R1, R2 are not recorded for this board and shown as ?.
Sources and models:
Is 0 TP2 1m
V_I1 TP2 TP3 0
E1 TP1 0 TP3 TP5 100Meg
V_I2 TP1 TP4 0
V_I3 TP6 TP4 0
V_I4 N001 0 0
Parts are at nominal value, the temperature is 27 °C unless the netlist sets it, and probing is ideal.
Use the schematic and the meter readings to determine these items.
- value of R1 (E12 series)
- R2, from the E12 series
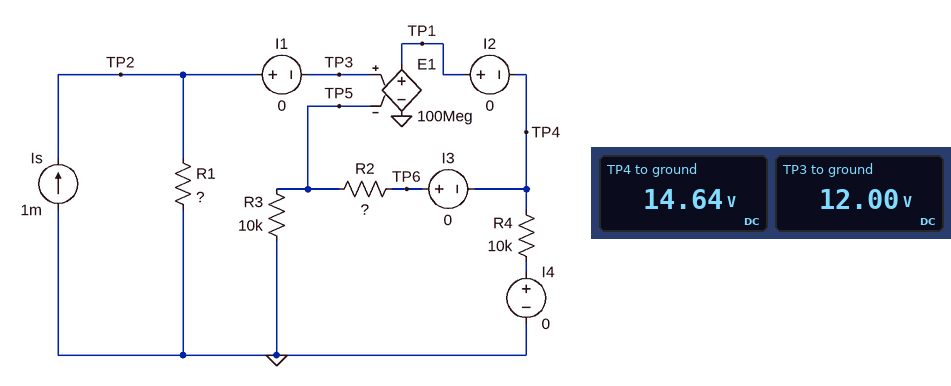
12 kΩ
2.2 kΩ
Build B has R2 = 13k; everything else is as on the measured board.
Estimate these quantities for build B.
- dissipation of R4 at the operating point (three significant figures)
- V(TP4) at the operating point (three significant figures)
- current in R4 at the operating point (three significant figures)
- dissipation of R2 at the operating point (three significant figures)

76.2 mW
27.6 V
2.76 mA
18.7 mW
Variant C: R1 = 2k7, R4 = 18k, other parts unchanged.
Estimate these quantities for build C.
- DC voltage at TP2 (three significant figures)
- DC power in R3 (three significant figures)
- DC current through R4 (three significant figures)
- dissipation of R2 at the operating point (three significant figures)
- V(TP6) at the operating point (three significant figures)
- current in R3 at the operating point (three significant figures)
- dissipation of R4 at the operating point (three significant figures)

2.70 V
729 µW
183 µA
160 µW
3.29 V
270 µA
603 µW
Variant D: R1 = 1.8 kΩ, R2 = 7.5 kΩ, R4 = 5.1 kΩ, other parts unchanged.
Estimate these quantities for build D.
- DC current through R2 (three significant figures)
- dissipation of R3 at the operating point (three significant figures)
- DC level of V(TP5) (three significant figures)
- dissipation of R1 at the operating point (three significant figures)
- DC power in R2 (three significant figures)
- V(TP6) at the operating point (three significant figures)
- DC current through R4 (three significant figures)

180 µA
324 µW
1.80 V
1.80 mW
243 µW
3.15 V
618 µA
